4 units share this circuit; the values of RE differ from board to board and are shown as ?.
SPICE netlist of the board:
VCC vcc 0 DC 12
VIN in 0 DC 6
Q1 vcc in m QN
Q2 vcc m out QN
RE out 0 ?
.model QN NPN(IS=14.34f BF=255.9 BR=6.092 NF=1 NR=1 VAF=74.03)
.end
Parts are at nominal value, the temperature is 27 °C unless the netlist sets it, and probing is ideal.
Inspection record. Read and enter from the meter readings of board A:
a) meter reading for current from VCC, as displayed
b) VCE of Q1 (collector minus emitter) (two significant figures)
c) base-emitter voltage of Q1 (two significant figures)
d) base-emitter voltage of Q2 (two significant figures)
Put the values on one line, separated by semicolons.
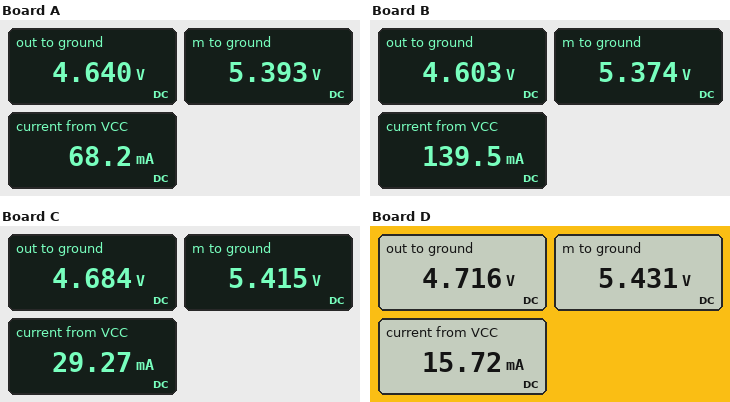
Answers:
68.2 mA; 6.6 V; 610 mV; 750 mV
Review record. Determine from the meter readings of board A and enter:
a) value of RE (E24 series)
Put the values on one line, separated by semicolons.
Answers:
68 Ω
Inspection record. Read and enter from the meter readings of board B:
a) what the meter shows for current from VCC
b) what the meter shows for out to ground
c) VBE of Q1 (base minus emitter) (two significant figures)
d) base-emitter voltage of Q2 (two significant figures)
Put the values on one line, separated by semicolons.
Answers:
139.5 mA; 4.603 V; 630 mV; 770 mV
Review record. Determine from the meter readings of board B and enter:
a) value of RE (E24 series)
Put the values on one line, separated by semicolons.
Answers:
33 Ω
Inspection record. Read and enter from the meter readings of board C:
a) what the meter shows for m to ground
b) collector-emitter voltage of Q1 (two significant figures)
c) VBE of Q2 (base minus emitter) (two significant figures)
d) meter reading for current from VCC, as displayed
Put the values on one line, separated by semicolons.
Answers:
5.415 V; 6.6 V; 730 mV; 29.27 mA
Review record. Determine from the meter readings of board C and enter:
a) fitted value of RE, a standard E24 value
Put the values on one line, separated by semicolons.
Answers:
160 Ω
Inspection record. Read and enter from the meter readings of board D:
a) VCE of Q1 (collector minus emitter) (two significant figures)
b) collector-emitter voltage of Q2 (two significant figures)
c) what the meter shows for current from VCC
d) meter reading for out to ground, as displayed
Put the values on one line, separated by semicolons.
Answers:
6.6 V; 7.3 V; 15.72 mA; 4.716 V
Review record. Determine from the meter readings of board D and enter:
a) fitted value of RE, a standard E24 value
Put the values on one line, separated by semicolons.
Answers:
300 Ω
